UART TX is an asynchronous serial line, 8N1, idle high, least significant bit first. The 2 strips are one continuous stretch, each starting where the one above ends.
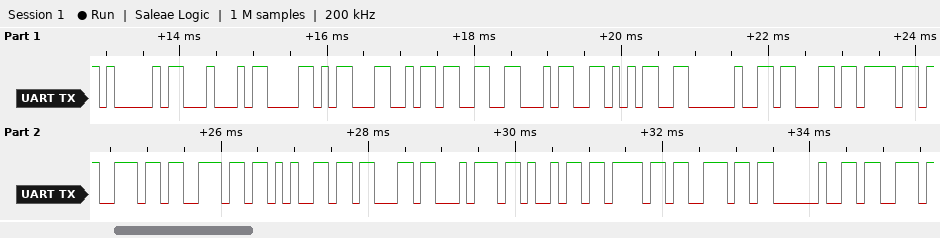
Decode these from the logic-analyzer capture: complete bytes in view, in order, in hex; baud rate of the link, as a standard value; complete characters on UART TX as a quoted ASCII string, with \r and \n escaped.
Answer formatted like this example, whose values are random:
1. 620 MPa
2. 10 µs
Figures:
1. 41 44 58 4C 33 34 35 20 63 6F 6E 6E 65 63 74 69 6F 6E 20 73
2. 9600 baud
3. "ADXL345 connection s"
